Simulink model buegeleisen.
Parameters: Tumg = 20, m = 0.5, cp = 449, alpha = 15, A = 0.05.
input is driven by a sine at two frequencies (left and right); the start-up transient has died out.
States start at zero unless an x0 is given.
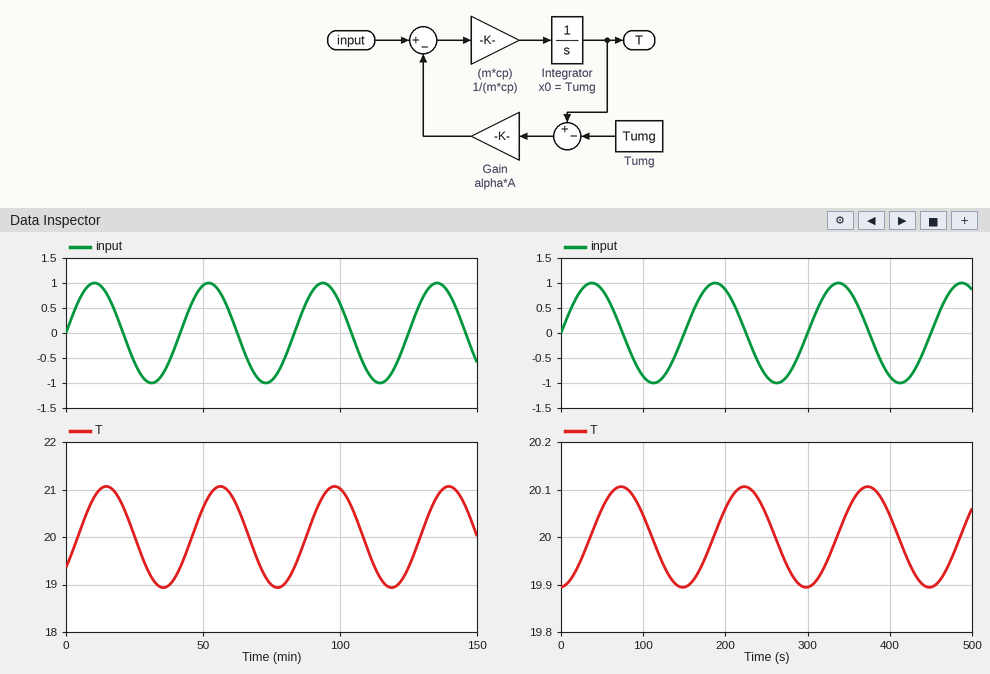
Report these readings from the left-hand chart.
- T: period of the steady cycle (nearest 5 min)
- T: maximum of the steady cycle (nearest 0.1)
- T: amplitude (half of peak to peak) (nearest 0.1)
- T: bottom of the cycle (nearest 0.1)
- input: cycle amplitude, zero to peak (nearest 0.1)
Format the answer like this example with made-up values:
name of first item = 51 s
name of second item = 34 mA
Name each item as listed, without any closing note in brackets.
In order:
T: period of the steady cycle = 40 min
T: maximum of the steady cycle = 21.1
T: amplitude (half of peak to peak) = 1.1
T: bottom of the cycle = 18.9
input: cycle amplitude, zero to peak = 1.0
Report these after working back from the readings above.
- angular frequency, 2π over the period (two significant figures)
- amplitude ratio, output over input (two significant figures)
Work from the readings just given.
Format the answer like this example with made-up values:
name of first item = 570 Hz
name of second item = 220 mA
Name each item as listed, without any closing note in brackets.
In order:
angular frequency, 2π over the period = 0.16 rad/min
amplitude ratio, output over input = 1.1
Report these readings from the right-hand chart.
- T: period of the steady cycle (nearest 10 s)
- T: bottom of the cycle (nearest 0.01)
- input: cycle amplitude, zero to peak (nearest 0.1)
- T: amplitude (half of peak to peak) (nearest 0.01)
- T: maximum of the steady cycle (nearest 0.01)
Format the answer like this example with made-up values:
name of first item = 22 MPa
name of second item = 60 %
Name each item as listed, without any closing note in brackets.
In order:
T: period of the steady cycle = 150 s
T: bottom of the cycle = 19.89
input: cycle amplitude, zero to peak = 1.0
T: amplitude (half of peak to peak) = 0.11
T: maximum of the steady cycle = 20.11
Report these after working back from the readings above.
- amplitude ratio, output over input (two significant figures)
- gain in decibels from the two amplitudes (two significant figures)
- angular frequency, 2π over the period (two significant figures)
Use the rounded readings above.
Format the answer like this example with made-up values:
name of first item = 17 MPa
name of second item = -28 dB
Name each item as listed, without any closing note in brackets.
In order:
amplitude ratio, output over input = 0.11
gain in decibels from the two amplitudes = -19 dB
angular frequency, 2π over the period = 0.042 rad/s
